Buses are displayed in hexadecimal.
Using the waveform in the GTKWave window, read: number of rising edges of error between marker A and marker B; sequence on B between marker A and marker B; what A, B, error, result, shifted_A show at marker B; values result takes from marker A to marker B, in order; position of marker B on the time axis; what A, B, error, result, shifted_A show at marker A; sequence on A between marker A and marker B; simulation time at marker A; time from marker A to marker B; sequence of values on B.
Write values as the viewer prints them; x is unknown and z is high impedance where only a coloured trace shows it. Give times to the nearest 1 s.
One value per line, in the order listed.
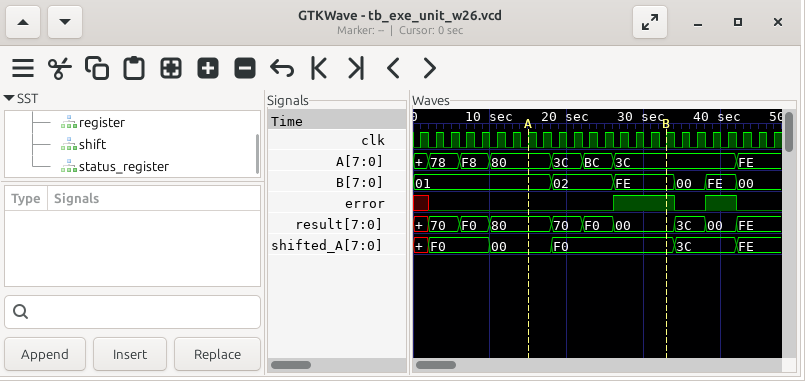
1
01, 02, FE
A=3C, B=FE, error=1, result=00, shifted_A=F0
80, 70, F0, 00
33 s
A=80, B=01, error=0, result=80, shifted_A=00
80, 3C, BC, 3C
15 s
18 s
01, 02, FE, 00, FE, 00
